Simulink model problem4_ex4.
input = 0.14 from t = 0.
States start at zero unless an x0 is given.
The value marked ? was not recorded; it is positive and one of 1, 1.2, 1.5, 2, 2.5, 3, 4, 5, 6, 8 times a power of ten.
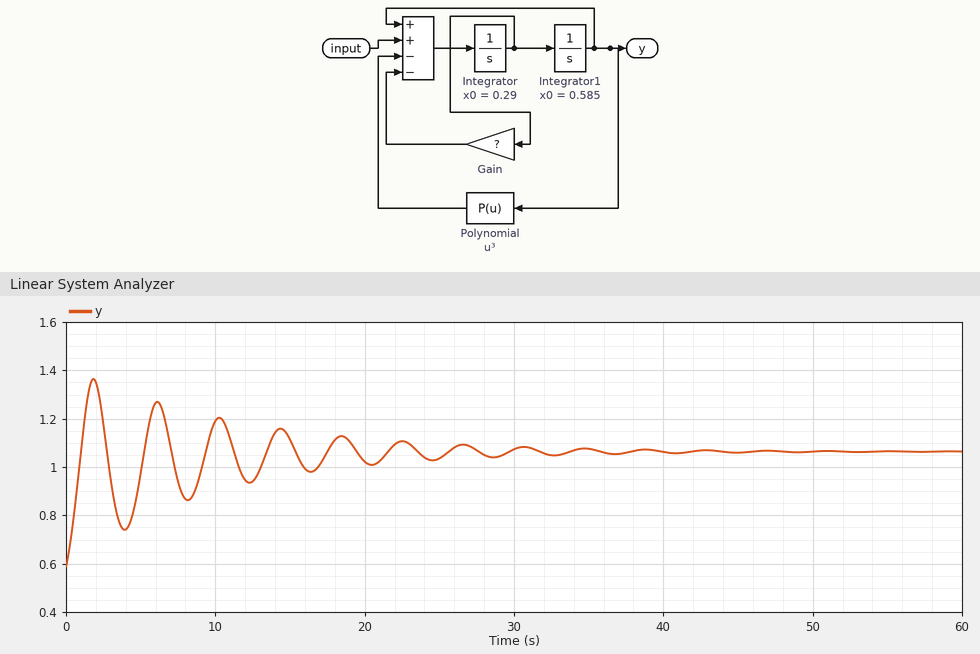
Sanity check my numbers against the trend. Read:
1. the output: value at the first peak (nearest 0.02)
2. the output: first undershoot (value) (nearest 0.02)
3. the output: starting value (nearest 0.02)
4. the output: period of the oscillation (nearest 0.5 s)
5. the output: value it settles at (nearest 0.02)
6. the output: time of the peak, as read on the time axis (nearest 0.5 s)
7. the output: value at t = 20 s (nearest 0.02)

1.36
0.74
0.58
4.5 s
1.06
2.0 s
1.02
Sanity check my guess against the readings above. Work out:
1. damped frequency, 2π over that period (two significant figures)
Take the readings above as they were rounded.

1.4 rad/s
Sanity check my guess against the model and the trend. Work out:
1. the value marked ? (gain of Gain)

0.2
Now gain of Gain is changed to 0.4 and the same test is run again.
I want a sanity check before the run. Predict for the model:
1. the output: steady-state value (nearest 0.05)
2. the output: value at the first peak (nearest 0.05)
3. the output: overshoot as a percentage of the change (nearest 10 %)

1.05
1.30
50 %
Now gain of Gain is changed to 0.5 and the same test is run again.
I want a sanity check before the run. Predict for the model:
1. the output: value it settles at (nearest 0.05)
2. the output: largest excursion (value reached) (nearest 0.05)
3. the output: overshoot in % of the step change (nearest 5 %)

1.05
1.30
45 %
